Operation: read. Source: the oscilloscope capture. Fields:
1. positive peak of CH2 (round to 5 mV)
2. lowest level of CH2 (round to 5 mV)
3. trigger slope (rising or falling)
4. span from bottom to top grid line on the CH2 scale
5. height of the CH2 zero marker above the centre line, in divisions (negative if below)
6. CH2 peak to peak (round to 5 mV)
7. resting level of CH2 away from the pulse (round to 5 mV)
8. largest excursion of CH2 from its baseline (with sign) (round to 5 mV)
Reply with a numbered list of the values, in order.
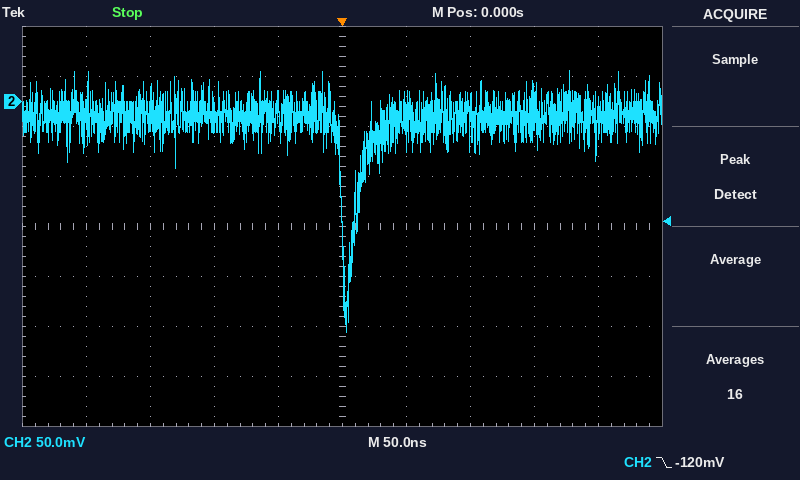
1. 30 mV
2. -230 mV
3. falling
4. 400 mV
5. +2.5 div
6. 260 mV
7. -15 mV
8. -215 mV
